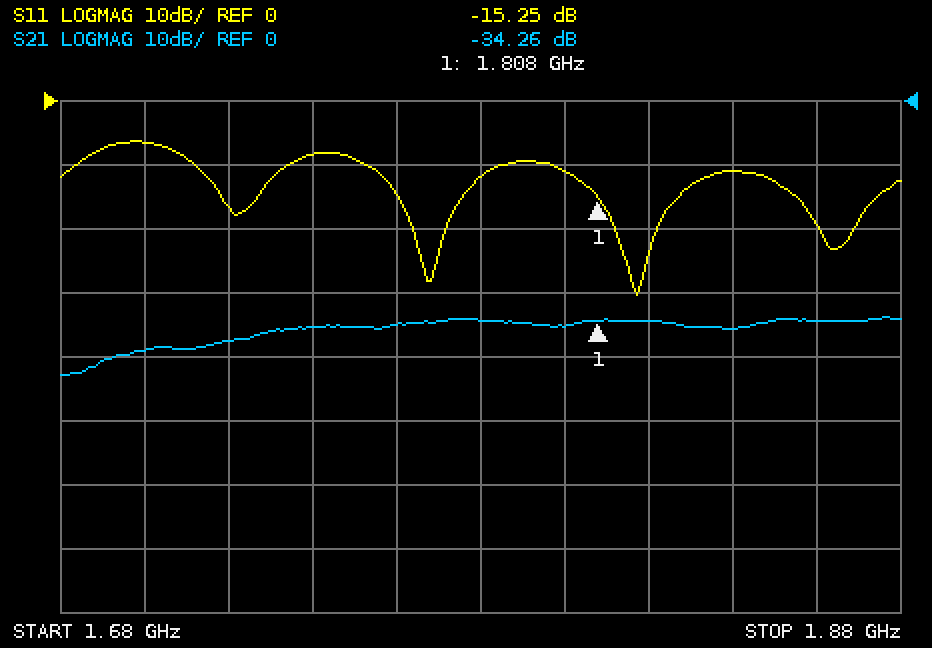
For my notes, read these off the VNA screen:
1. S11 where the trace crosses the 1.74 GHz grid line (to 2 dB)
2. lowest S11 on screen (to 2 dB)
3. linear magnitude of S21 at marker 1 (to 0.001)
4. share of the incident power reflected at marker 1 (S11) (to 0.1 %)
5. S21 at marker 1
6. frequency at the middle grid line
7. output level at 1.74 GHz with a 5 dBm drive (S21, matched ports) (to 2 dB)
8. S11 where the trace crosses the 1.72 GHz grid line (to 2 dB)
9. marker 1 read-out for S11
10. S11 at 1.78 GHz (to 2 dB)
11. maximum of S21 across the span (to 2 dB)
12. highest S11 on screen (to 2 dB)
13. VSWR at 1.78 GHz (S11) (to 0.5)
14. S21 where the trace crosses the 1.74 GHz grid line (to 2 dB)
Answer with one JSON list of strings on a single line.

["-8 dB", "-30 dB", "0.019", "3.0 %", "-34.26 dB", "1.78 GHz", "-30 dBm", "-16 dB", "-15.25 dB", "-12 dB", "-34 dB", "-6 dB", "1.5", "-36 dB"]
